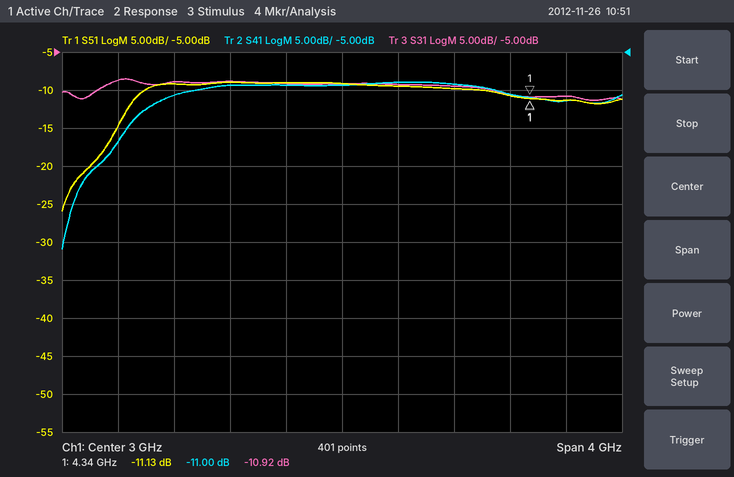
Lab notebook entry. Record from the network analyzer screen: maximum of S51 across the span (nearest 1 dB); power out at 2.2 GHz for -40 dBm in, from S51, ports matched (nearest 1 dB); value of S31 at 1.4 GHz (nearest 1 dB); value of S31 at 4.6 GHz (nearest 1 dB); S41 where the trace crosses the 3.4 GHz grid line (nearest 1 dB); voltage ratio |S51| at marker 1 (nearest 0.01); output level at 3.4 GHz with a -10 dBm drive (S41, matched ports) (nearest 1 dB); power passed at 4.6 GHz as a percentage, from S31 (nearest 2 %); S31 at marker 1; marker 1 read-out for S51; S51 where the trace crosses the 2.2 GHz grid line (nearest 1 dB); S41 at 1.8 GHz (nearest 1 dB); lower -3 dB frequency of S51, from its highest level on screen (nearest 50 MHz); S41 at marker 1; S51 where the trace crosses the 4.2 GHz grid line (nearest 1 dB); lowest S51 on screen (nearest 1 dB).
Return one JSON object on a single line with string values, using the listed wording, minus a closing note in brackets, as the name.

{"maximum of S51 across the span": "-9 dB", "power out at 2.2 GHz for -40 dBm in, from S51, ports matched": "-49 dBm", "value of S31 at 1.4 GHz": "-9 dB", "value of S31 at 4.6 GHz": "-11 dB", "S41 where the trace crosses the 3.4 GHz grid line": "-9 dB", "voltage ratio |S51| at marker 1": "0.28", "output level at 3.4 GHz with a -10 dBm drive (S41, matched ports)": "-19 dBm", "power passed at 4.6 GHz as a percentage, from S31": "8 %", "S31 at marker 1": "-10.92 dB", "marker 1 read-out for S51": "-11.13 dB", "S51 where the trace crosses the 2.2 GHz grid line": "-9 dB", "S41 at 1.8 GHz": "-11 dB", "lower -3 dB frequency of S51, from its highest level on screen": "1.50 GHz", "S41 at marker 1": "-11.00 dB", "S51 where the trace crosses the 4.2 GHz grid line": "-11 dB", "lowest S51 on screen": "-26 dB"}
